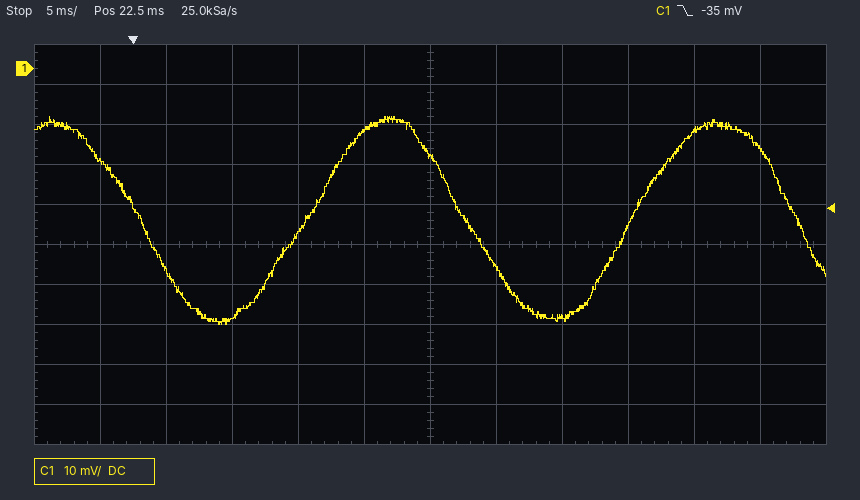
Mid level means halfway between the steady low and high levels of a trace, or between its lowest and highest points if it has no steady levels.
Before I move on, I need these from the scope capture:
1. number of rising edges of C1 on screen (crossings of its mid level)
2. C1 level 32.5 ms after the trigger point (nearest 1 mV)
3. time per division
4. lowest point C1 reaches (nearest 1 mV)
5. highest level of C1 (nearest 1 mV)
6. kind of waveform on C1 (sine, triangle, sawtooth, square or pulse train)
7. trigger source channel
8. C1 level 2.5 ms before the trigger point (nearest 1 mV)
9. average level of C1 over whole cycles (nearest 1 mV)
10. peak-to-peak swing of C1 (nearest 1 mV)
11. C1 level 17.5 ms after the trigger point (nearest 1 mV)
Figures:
2
-62 mV
5 ms
-64 mV
-12 mV
sine
C1
-23 mV
-38 mV
52 mV
-15 mV
